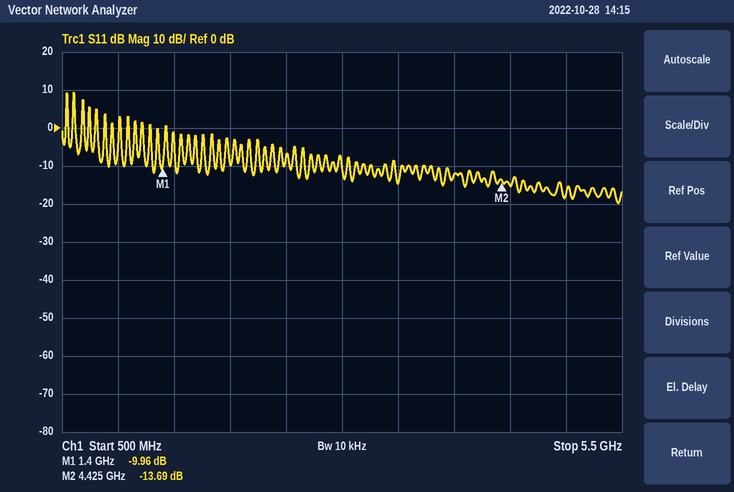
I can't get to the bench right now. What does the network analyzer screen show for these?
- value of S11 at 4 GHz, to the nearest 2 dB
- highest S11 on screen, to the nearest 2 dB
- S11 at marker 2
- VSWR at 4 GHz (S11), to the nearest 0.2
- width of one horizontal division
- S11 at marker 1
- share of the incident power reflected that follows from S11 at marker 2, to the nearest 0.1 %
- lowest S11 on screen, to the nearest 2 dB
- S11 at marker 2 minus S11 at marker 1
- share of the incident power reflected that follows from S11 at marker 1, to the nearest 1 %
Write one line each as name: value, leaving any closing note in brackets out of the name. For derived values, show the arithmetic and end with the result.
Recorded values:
value of S11 at 4 GHz, to the nearest 2 dB: -12 dB
highest S11 on screen, to the nearest 2 dB: 10 dB
S11 at marker 2: -13.69 dB
VSWR at 4 GHz (S11), to the nearest 0.2: |Γ| = 10^(-12/20) = 0.2512; VSWR = (1 + 0.2512)/(1 − 0.2512) ≈ 1.67, so 1.6 to the nearest 0.2
width of one horizontal division: 500 MHz
S11 at marker 1: -9.96 dB
share of the incident power reflected that follows from S11 at marker 2, to the nearest 0.1 %: 10^(-13.69/10) ≈ 4.3 %
lowest S11 on screen, to the nearest 2 dB: -20 dB
S11 at marker 2 minus S11 at marker 1: -13.69 − (-9.96) = -3.73 dB
share of the incident power reflected that follows from S11 at marker 1, to the nearest 1 %: 10^(-9.96/10) ≈ 10 %
